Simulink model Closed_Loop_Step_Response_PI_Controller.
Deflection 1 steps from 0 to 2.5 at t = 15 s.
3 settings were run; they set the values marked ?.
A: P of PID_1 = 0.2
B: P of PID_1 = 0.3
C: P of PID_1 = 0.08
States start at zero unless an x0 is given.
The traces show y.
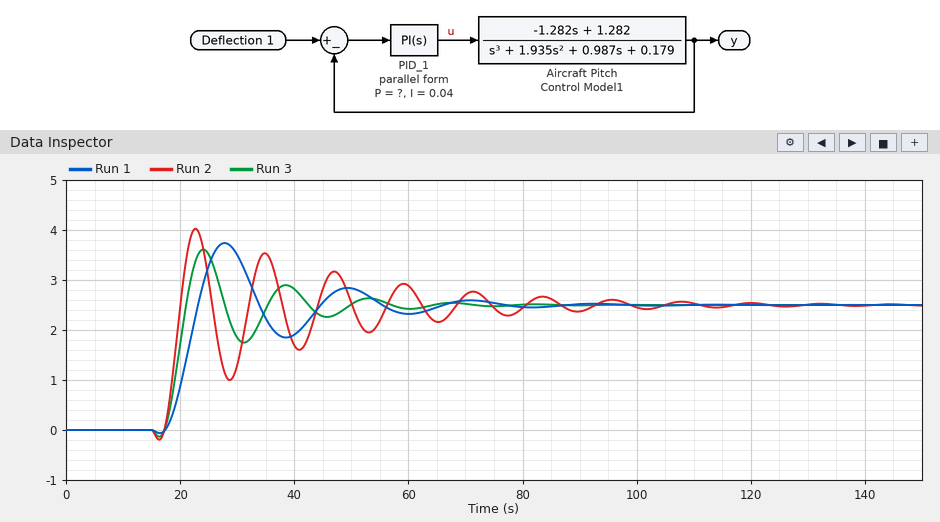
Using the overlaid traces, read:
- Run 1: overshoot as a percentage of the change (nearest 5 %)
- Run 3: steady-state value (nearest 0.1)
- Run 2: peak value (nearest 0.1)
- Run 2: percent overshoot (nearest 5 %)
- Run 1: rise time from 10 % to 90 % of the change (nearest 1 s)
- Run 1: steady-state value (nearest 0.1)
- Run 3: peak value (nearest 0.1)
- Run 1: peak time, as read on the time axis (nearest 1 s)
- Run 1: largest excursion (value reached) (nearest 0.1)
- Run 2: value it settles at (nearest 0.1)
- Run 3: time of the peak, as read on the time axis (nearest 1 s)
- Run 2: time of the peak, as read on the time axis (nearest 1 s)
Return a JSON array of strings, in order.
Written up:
["50 %", "2.5", "4.0", "60 %", "4 s", "2.5", "3.6", "28 s", "3.7", "2.5", "24 s", "23 s"]
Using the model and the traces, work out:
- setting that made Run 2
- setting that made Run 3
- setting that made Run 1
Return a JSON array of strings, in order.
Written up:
["B", "A", "C"]
